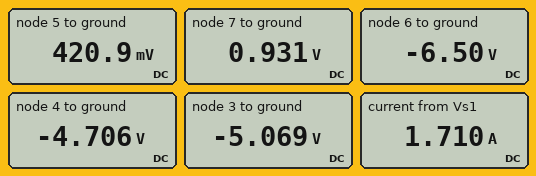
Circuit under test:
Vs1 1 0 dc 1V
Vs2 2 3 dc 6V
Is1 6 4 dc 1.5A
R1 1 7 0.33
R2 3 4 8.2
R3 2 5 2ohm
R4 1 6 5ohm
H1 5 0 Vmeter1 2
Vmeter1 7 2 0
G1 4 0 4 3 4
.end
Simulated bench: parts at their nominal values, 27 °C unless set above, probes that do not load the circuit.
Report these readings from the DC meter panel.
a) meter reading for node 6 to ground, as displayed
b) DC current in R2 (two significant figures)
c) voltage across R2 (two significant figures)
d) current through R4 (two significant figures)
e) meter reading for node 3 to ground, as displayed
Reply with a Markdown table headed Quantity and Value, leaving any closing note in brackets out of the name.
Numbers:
| Quantity | Value |
|---|---|
| meter reading for node 6 to ground, as displayed | -6.50 V |
| DC current in R2 | 44 mA |
| voltage across R2 | 360 mV |
| current through R4 | 1.5 A |
| meter reading for node 3 to ground, as displayed | -5.069 V |
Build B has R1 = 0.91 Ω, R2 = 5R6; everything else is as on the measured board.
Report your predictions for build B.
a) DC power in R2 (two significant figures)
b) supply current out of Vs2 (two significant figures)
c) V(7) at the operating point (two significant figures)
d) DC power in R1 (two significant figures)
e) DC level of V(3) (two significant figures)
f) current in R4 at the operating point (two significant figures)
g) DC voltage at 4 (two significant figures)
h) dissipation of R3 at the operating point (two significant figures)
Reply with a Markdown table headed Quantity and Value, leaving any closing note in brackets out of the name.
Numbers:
| Quantity | Value |
|---|---|
| DC power in R2 | 23 mW |
| supply current out of Vs2 | 64 mA |
| V(7) at the operating point | 840 mV |
| DC power in R1 | 29 mW |
| DC level of V(3) | -5.2 V |
| current in R4 at the operating point | 1.5 A |
| DC voltage at 4 | -4.8 V |
| dissipation of R3 at the operating point | 120 mW |
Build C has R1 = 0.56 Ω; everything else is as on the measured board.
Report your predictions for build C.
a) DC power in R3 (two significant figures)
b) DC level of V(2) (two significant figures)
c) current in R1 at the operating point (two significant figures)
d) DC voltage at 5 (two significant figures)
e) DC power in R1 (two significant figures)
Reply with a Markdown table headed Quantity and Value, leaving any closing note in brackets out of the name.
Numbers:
| Quantity | Value |
|---|---|
| DC power in R3 | 120 mW |
| DC level of V(2) | 890 mV |
| current in R1 at the operating point | 200 mA |
| DC voltage at 5 | 400 mV |
| DC power in R1 | 22 mW |
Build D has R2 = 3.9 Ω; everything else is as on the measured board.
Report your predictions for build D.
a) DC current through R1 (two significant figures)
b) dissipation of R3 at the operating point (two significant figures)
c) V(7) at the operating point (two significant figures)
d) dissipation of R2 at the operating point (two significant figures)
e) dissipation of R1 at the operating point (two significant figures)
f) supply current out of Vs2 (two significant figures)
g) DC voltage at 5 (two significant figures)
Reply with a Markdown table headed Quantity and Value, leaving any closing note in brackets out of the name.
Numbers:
| Quantity | Value |
|---|---|
| DC current through R1 | 190 mA |
| dissipation of R3 at the operating point | 160 mW |
| V(7) at the operating point | 940 mV |
| dissipation of R2 at the operating point | 32 mW |
| dissipation of R1 at the operating point | 12 mW |
| supply current out of Vs2 | 90 mA |
| DC voltage at 5 | 380 mV |
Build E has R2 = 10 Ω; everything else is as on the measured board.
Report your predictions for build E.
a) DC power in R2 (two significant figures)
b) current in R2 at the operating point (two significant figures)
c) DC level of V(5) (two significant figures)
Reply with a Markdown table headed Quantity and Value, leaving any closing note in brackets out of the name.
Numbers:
| Quantity | Value |
|---|---|
| DC power in R2 | 13 mW |
| current in R2 at the operating point | 37 mA |
| DC level of V(5) | 430 mV |
